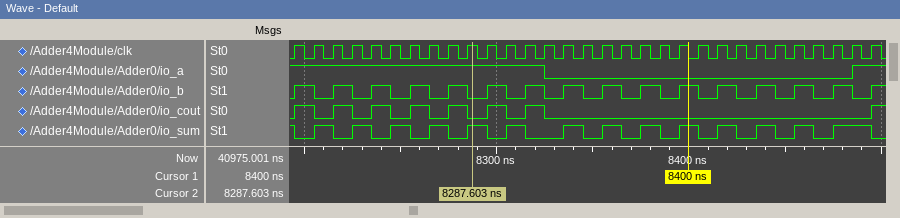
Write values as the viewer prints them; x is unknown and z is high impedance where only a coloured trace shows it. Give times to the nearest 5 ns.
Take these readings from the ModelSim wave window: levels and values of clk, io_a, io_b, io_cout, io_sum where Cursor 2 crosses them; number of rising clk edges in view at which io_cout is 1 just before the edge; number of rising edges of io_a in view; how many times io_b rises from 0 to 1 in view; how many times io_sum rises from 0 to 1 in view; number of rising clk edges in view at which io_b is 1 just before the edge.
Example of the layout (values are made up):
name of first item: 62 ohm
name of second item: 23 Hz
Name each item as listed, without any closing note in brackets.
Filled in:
levels and values of clk, io_a, io_b, io_cout, io_sum where Cursor 2 crosses them: clk=1, io_a=1, io_b=0, io_cout=0, io_sum=1
number of rising clk edges in view at which io_cout is 1 just before the edge: 7
number of rising edges of io_a in view: 1
how many times io_b rises from 0 to 1 in view: 16
how many times io_sum rises from 0 to 1 in view: 14
number of rising clk edges in view at which io_b is 1 just before the edge: 15
